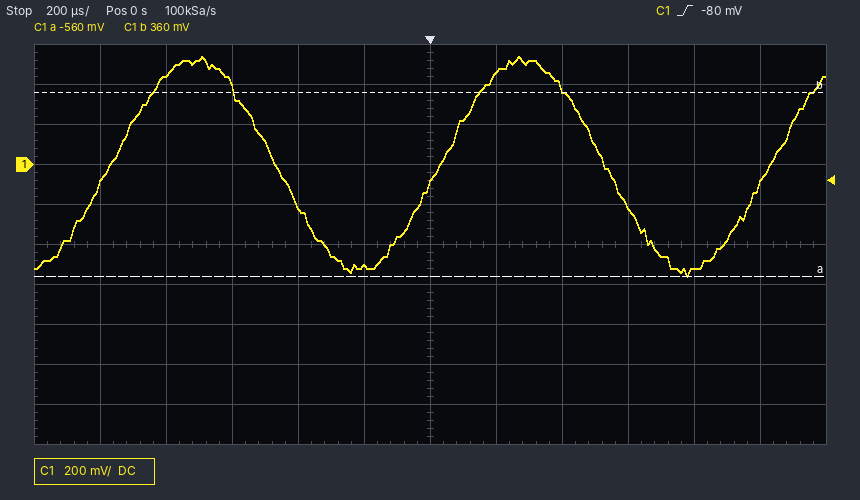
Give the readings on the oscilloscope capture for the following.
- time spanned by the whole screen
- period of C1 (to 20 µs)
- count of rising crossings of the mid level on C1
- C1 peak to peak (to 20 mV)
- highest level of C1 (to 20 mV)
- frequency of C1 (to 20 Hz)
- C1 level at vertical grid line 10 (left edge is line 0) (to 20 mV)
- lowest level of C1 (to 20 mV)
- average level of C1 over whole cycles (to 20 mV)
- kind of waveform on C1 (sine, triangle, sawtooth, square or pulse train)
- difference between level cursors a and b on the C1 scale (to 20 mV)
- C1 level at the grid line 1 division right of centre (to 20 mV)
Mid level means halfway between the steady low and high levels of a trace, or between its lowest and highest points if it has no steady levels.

2.4 ms
1.00 ms
3
1.10 V
540 mV
1.00 kHz
-520 mV
-560 mV
0 mV
sine
920 mV
460 mV
